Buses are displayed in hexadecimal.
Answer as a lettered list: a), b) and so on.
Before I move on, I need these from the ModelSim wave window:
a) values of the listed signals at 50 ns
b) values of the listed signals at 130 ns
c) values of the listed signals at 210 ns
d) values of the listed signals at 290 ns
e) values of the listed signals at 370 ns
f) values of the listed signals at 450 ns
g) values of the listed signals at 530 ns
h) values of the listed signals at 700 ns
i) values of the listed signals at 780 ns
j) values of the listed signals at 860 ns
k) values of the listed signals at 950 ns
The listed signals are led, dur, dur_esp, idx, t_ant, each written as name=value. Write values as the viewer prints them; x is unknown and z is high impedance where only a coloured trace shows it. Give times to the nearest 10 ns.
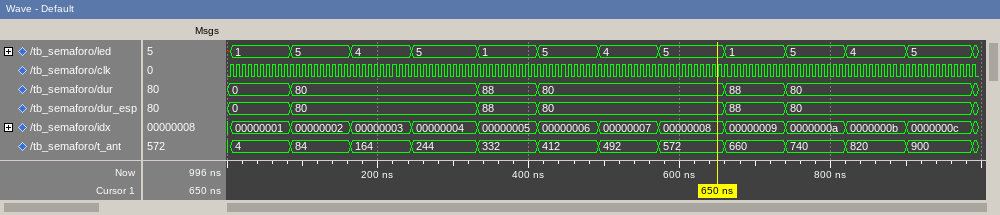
a) led=1, dur=0, dur_esp=0, idx=00000001, t_ant=4
b) led=5, dur=80, dur_esp=80, idx=00000002, t_ant=84
c) led=4, dur=80, dur_esp=80, idx=00000003, t_ant=164
d) led=5, dur=80, dur_esp=80, idx=00000004, t_ant=244
e) led=1, dur=88, dur_esp=88, idx=00000005, t_ant=332
f) led=5, dur=80, dur_esp=80, idx=00000006, t_ant=412
g) led=4, dur=80, dur_esp=80, idx=00000007, t_ant=492
h) led=1, dur=88, dur_esp=88, idx=00000009, t_ant=660
i) led=5, dur=80, dur_esp=80, idx=0000000a, t_ant=740
j) led=4, dur=80, dur_esp=80, idx=0000000b, t_ant=820
k) led=5, dur=80, dur_esp=80, idx=0000000c, t_ant=900
